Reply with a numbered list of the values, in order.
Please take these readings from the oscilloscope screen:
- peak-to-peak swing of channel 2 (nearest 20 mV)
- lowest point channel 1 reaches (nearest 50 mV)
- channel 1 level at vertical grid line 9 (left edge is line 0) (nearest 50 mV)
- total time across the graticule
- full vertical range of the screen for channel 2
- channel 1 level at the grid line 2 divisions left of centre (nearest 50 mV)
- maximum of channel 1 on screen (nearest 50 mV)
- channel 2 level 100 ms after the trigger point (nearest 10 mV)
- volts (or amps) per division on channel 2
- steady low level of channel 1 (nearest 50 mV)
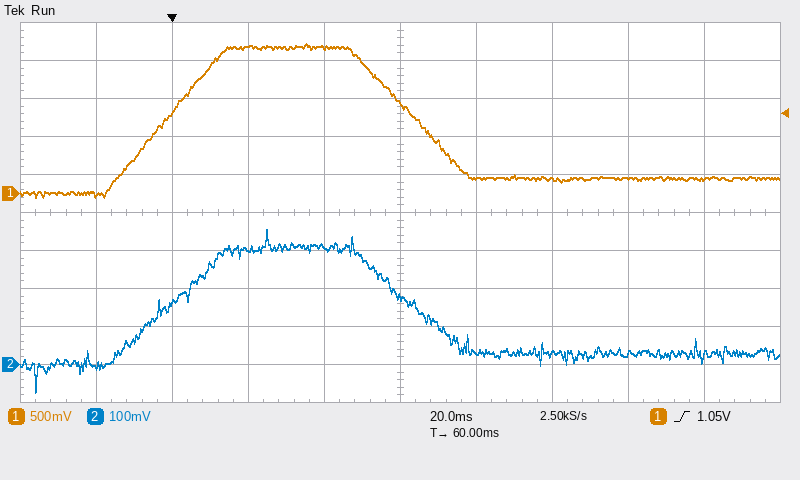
1. 420 mV
2. -50 mV
3. 200 mV
4. 200 ms
5. 1 V
6. 1.95 V
7. 1.95 V
8. 30 mV
9. 100 mV
10. 200 mV
